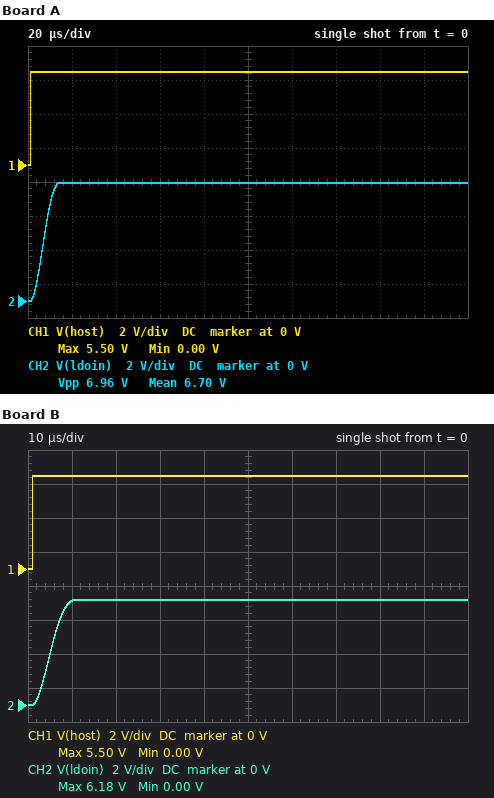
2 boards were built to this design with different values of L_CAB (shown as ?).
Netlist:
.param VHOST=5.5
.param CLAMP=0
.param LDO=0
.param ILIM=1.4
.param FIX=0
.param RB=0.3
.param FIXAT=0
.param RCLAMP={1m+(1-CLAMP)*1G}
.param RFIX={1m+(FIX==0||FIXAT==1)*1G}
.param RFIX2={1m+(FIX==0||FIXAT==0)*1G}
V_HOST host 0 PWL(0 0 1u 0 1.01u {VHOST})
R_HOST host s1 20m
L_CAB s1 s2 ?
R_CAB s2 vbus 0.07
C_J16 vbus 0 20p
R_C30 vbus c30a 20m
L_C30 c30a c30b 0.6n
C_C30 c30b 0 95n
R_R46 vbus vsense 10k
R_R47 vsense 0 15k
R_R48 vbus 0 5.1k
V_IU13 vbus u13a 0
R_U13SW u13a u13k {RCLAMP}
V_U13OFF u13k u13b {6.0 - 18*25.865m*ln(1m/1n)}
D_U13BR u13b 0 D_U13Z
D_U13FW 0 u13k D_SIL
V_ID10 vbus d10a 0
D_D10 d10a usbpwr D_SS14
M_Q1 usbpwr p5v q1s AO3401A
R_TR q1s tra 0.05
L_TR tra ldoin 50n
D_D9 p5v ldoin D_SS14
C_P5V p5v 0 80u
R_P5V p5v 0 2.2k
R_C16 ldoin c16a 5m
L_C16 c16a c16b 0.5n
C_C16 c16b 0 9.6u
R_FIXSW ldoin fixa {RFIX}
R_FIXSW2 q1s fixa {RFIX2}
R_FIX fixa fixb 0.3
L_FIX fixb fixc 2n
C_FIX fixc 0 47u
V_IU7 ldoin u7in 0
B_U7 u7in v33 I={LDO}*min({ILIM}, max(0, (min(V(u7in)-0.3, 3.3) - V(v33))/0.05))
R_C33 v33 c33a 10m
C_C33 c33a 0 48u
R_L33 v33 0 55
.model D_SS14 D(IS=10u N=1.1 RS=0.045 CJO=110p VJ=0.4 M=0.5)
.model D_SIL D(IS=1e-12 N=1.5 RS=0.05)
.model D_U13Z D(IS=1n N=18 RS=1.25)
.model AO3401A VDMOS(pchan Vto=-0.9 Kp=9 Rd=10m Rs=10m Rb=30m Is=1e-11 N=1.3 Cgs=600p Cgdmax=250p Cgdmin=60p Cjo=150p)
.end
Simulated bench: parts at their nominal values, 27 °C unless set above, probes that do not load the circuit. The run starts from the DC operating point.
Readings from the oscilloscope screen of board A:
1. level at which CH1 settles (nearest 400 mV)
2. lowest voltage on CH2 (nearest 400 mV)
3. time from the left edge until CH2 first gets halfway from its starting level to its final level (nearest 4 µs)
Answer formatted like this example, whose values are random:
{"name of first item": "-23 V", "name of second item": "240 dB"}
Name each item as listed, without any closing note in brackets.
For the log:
{"level at which CH1 settles": "5.6 V", "lowest voltage on CH2": "0 V", "time from the left edge until CH2 first gets halfway from its starting level to its final level": "8 µs"}
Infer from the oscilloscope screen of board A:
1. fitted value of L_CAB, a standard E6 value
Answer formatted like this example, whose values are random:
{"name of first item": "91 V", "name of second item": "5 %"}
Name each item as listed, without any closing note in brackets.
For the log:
{"fitted value of L_CAB, a standard E6 value": "1.5 µH"}
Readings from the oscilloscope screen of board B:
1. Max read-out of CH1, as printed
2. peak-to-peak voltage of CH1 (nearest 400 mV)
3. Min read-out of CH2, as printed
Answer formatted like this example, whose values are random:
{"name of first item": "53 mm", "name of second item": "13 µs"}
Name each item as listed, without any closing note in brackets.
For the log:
{"Max read-out of CH1, as printed": "5.50 V", "peak-to-peak voltage of CH1": "5.6 V", "Min read-out of CH2, as printed": "0.00 V"}
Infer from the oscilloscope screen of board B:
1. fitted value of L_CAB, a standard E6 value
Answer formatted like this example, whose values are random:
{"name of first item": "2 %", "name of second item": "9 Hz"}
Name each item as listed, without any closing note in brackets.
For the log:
{"fitted value of L_CAB, a standard E6 value": "680 nH"}
